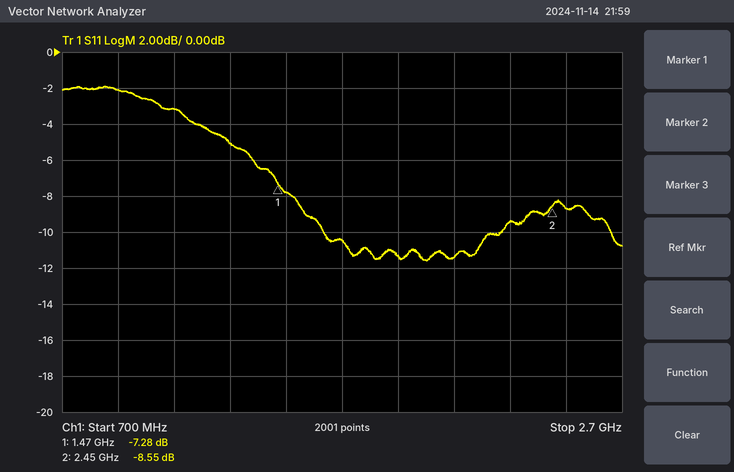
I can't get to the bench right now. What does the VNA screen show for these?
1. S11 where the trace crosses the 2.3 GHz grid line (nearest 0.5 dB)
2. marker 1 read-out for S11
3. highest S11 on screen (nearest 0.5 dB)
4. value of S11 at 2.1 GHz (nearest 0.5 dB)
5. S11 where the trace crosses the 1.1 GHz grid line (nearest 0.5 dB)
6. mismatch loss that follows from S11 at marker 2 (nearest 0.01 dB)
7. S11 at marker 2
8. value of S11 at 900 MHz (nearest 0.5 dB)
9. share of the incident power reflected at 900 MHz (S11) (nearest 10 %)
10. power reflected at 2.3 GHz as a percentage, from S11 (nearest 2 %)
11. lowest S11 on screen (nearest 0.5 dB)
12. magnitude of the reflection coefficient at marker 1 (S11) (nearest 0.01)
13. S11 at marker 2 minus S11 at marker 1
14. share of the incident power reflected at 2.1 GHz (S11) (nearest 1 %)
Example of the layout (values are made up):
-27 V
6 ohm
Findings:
-9.5 dB
-7.28 dB
-2.0 dB
-11.5 dB
-3.0 dB
0.65 dB
-8.55 dB
-2.0 dB
60 %
12 %
-11.5 dB
0.43
-1.27 dB
7 %
